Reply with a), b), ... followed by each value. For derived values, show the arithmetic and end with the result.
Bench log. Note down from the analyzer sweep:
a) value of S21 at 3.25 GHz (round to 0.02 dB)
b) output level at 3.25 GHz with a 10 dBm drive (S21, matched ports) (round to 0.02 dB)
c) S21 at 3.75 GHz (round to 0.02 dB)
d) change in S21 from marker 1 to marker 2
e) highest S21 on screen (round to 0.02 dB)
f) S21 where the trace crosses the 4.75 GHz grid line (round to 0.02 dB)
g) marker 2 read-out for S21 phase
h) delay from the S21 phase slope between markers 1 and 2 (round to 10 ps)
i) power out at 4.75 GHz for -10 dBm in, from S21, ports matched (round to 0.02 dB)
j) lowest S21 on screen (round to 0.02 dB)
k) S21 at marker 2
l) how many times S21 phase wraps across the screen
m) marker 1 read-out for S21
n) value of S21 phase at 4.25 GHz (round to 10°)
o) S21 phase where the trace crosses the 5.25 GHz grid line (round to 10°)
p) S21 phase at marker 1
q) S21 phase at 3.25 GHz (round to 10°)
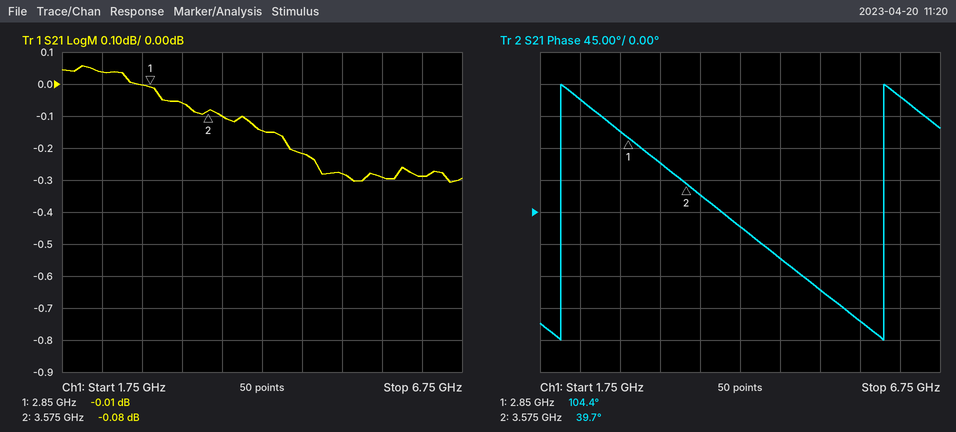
a) -0.06 dB
b) 10 dBm + (-0.06 dB) = 9.94 dBm
c) -0.10 dB
d) -0.08 − (-0.01) = -0.07 dB
e) 0.06 dB
f) -0.22 dB
g) 39.7°
h) −(39.7° − (104.4°))/(360° × 725 MHz) ≈ 248 ps, so 250 ps to the nearest 10 ps
i) -10 dBm + (-0.22 dB) = -10.22 dBm
j) -0.30 dB
k) -0.08 dB
l) 2
m) -0.01 dB
n) -20°
o) -110°
p) 104.4°
q) 70°
